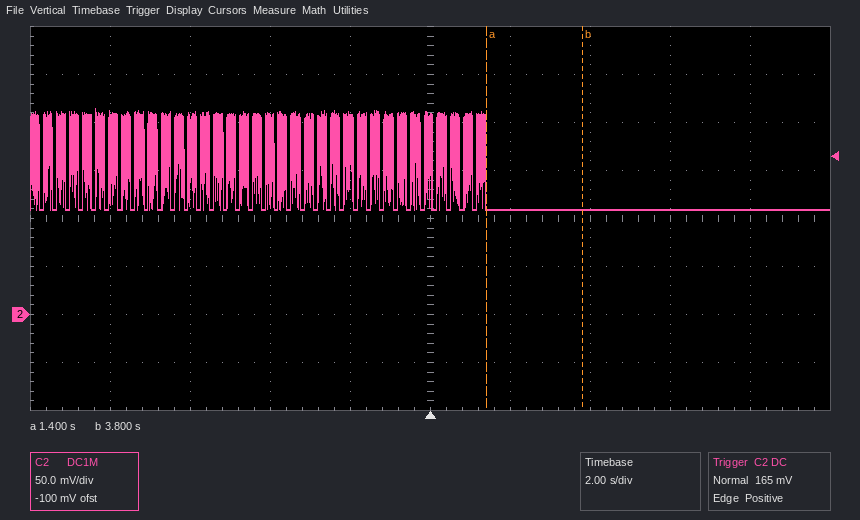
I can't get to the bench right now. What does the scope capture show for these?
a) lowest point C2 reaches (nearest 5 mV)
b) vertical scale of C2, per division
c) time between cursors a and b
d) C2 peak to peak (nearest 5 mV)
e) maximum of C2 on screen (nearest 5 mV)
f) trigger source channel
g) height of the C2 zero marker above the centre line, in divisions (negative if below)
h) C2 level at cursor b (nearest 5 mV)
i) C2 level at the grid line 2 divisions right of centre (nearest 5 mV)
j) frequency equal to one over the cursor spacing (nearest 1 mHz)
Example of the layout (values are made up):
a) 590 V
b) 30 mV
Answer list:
a) 110 mV
b) 50 mV
c) 2.4 s
d) 105 mV
e) 215 mV
f) C2
g) -2.0 div
h) 110 mV
i) 110 mV
j) 417 mHz
